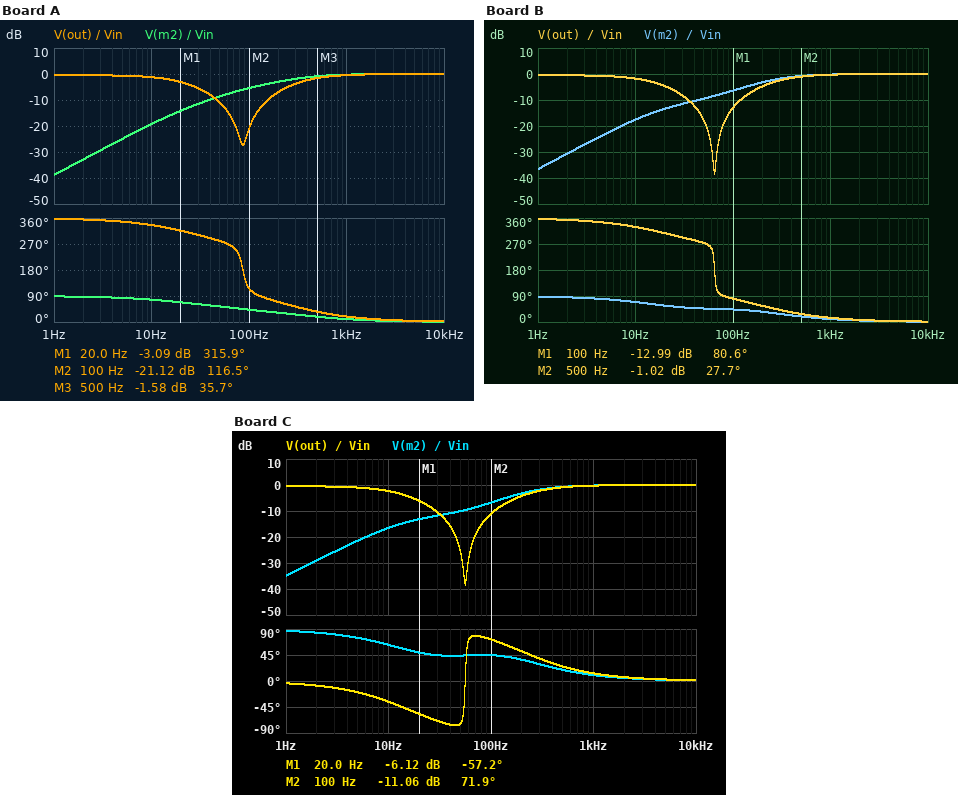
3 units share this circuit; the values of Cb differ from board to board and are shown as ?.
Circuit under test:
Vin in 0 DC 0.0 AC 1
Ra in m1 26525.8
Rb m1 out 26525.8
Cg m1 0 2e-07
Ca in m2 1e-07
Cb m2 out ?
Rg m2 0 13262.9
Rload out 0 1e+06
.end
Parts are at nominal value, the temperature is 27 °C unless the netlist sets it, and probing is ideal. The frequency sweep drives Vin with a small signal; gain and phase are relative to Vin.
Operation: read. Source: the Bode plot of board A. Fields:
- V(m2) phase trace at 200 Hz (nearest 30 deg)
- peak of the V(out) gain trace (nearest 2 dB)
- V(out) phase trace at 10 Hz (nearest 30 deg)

30 deg
0 dB
330 deg
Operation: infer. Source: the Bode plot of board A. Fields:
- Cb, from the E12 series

39 nF
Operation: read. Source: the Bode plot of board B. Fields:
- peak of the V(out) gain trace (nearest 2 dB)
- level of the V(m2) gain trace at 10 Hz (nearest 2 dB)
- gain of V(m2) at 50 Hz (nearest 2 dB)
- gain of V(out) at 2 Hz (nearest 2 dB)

0 dB
-18 dB
-10 dB
0 dB
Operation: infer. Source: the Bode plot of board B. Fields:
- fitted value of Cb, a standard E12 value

82 nF
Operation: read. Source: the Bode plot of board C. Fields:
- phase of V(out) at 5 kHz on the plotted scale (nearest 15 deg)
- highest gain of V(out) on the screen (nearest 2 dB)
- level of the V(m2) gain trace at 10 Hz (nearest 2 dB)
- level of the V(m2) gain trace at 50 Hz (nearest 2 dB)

0 deg
0 dB
-16 dB
-10 dB
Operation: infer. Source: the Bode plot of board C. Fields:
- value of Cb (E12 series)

120 nF
